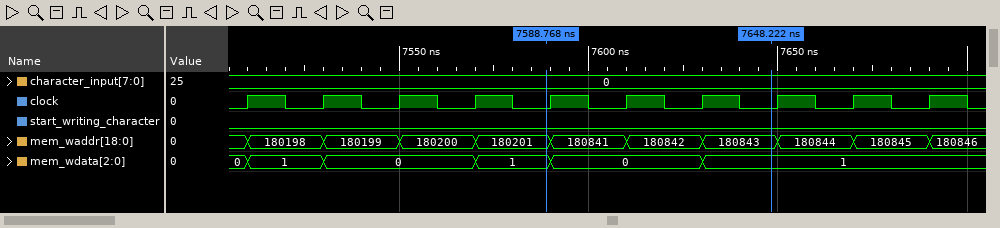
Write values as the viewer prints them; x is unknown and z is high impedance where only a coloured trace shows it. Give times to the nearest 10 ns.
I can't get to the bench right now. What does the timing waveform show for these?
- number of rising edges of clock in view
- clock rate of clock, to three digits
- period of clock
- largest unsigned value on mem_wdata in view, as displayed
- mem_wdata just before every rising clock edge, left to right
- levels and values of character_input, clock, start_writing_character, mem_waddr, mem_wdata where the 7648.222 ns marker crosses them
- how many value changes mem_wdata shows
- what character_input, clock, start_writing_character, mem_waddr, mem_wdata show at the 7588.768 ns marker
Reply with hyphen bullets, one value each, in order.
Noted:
- 10
- 50.0 MHz
- 20 ns
- 1
- 0, 1, 0, 0, 1, 0, 0, 1, 1, 1
- character_input=0, clock=0, start_writing_character=0, mem_waddr=180843, mem_wdata=1
- 5
- character_input=0, clock=0, start_writing_character=0, mem_waddr=180201, mem_wdata=1
